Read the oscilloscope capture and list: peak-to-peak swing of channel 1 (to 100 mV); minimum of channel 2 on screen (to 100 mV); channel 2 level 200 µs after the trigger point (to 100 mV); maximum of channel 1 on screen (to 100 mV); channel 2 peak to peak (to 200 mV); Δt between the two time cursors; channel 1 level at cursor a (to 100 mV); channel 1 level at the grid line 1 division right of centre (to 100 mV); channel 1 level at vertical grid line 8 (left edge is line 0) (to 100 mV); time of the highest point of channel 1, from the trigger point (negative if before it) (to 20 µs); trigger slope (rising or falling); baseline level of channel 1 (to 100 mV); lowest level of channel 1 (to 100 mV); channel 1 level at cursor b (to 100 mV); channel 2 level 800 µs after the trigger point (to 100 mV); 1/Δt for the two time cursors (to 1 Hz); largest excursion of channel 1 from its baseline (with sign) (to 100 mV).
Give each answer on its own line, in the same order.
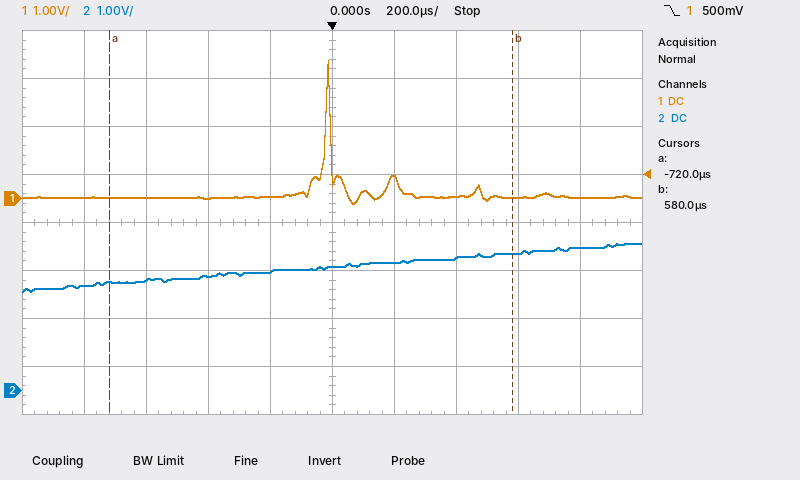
3.0 V
2.1 V
2.7 V
2.9 V
1.0 V
1.30 ms
0.0 V
400 mV
0.0 V
-20 µs
falling
0.0 V
-100 mV
0.0 V
3.0 V
769 Hz
+2.9 V
